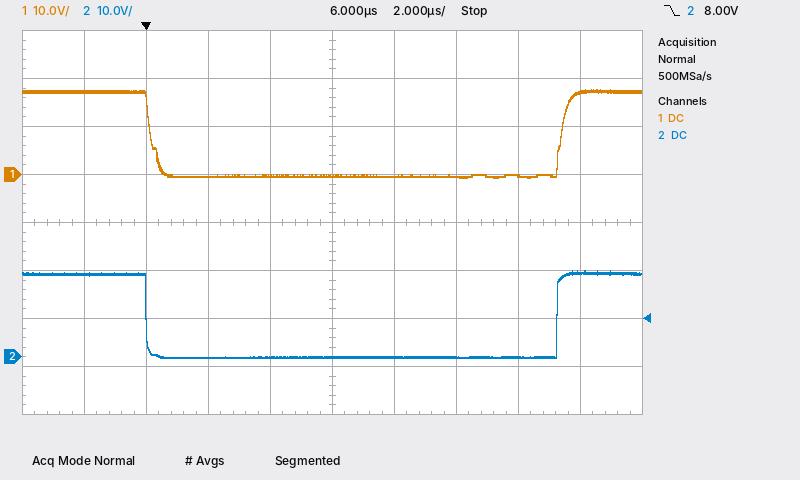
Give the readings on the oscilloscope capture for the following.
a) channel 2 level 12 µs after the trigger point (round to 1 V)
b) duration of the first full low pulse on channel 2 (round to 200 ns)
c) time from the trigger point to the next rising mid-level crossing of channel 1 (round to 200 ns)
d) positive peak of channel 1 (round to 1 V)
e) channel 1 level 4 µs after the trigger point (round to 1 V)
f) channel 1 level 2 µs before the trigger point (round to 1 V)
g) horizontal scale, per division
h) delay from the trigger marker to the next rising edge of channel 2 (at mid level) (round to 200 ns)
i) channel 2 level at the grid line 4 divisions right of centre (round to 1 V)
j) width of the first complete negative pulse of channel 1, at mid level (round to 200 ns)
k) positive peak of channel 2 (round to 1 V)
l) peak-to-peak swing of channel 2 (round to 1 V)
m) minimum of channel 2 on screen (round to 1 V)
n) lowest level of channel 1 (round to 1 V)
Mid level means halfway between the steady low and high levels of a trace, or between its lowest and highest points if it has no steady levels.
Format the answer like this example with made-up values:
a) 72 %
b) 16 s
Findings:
a) 0 V
b) 13.2 µs
c) 13.4 µs
d) 18 V
e) 0 V
f) 17 V
g) 2 µs
h) 13.2 µs
i) 18 V
j) 13.2 µs
k) 18 V
l) 18 V
m) 0 V
n) -1 V
